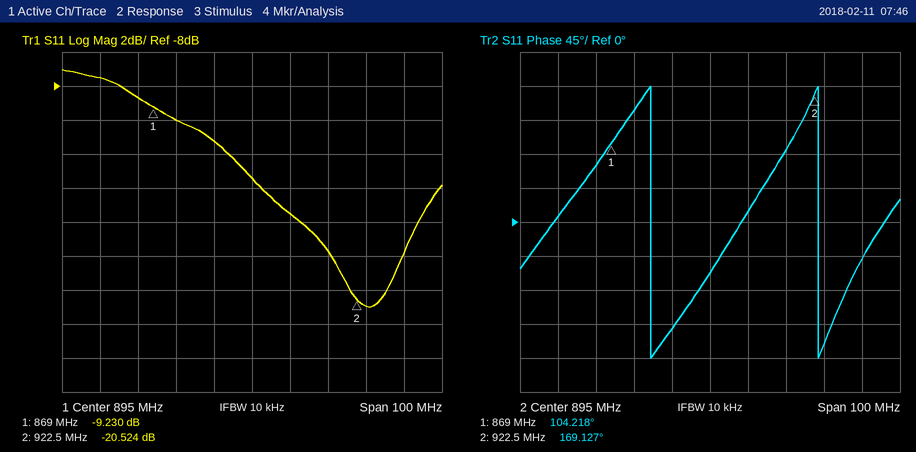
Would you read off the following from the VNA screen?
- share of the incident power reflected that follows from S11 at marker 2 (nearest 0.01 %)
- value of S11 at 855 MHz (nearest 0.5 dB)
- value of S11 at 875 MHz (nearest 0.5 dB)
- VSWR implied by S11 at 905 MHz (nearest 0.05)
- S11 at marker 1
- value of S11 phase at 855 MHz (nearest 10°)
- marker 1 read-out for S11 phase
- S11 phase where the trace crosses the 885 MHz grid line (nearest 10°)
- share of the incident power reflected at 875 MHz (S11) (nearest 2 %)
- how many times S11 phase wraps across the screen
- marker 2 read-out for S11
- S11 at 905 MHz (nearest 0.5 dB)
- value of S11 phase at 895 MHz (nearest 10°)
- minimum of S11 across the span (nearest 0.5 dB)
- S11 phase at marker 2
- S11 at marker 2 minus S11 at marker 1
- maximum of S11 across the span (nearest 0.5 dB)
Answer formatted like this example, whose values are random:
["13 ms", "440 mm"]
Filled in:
["0.89 %", "-7.5 dB", "-10.0 dB", "1.40", "-9.230 dB", "10°", "104.218°", "-140°", "10 %", "2", "-20.524 dB", "-15.5 dB", "-70°", "-21.0 dB", "169.127°", "-11.294 dB", "-7.0 dB"]
